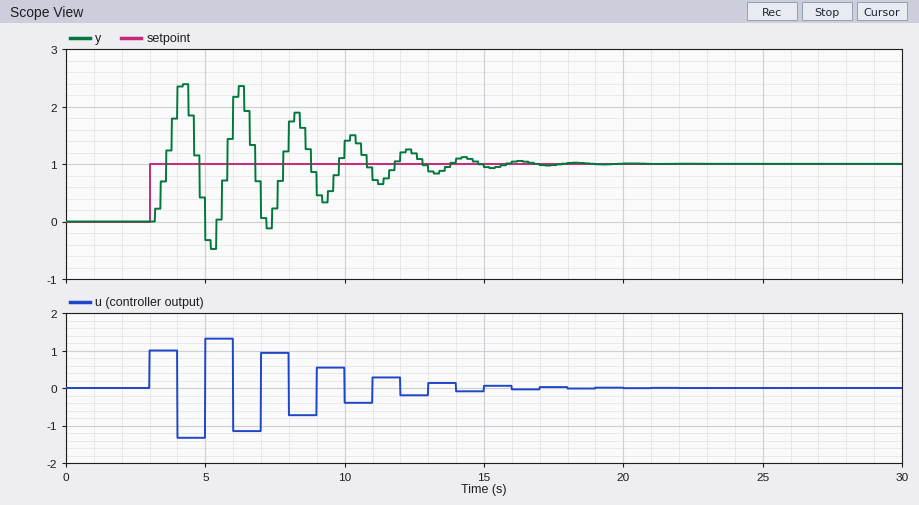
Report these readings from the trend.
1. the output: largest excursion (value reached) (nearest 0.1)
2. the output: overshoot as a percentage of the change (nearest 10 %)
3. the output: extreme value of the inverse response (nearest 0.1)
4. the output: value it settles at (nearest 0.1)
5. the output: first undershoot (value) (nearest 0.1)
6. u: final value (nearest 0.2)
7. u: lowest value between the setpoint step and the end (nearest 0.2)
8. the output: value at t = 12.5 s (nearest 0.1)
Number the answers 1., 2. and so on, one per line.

1. 2.4
2. 140 %
3. -0.5
4. 1.0
5. -0.5
6. 0.0
7. -1.4
8. 1.2
